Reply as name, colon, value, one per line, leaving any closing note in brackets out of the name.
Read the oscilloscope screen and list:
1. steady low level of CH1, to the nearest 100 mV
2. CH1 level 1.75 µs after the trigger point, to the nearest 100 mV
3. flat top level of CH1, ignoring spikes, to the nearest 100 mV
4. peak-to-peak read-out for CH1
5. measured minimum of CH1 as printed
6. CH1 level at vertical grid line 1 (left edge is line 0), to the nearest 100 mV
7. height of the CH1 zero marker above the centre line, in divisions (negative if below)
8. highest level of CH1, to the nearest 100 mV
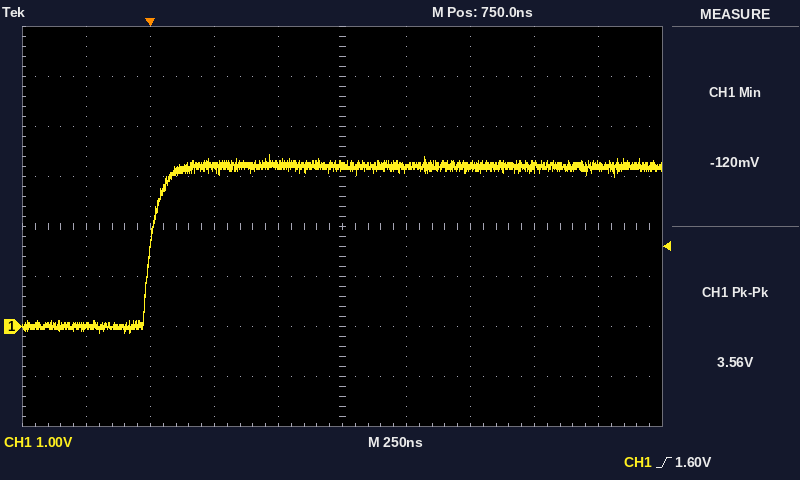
steady low level of CH1, to the nearest 100 mV: 0.0 V
CH1 level 1.75 µs after the trigger point, to the nearest 100 mV: 3.2 V
flat top level of CH1, ignoring spikes, to the nearest 100 mV: 3.2 V
peak-to-peak read-out for CH1: 3.56 V
measured minimum of CH1 as printed: -120 mV
CH1 level at vertical grid line 1 (left edge is line 0), to the nearest 100 mV: 0.0 V
height of the CH1 zero marker above the centre line, in divisions: -2.0 div
highest level of CH1, to the nearest 100 mV: 3.4 V
